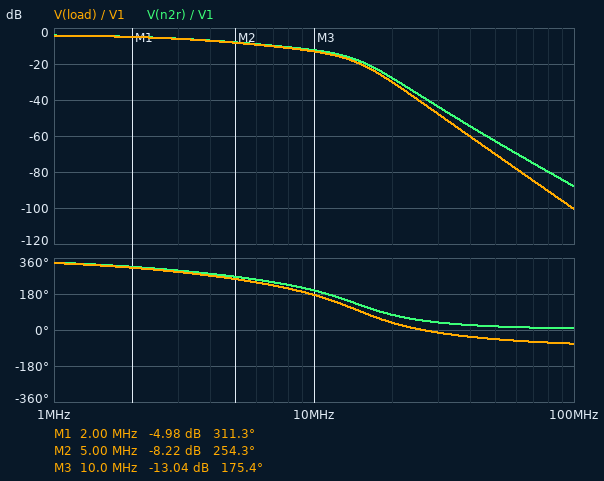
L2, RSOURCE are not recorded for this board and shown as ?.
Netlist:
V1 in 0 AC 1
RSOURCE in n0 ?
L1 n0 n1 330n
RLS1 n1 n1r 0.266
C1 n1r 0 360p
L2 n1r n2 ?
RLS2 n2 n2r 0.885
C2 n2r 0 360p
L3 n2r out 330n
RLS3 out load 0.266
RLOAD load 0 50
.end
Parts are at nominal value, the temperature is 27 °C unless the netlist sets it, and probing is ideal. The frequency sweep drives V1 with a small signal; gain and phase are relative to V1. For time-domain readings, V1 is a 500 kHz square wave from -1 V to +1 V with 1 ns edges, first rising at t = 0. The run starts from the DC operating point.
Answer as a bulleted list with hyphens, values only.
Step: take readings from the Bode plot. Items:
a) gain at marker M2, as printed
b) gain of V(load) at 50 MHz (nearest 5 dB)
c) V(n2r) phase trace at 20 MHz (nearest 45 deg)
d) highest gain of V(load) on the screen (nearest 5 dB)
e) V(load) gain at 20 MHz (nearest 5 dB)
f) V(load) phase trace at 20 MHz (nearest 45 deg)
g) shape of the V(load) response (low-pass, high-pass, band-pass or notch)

- -8.22 dB
- -70 dB
- 90 deg
- -5 dB
- -30 dB
- 45 deg
- low-pass
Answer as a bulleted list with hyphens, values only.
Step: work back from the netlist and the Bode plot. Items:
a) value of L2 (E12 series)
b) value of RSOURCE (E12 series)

- 3.9 µH
- 27 Ω
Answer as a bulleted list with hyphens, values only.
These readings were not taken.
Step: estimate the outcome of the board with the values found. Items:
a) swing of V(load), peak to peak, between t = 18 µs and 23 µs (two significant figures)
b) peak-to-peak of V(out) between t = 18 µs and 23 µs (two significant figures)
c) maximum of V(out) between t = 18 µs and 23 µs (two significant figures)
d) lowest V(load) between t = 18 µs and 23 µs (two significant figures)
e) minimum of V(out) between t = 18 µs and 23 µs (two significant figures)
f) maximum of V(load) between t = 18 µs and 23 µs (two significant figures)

- 1.3 V
- 1.3 V
- 640 mV
- -640 mV
- -640 mV
- 640 mV
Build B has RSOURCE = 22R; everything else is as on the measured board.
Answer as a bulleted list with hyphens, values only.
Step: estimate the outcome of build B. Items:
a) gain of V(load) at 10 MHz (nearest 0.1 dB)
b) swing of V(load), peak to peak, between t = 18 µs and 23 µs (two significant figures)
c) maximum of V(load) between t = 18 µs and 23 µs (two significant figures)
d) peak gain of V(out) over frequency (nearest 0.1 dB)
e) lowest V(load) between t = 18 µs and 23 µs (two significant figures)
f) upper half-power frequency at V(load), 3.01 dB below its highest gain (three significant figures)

- -12.4 dB
- 1.4 V
- 680 mV
- -3.3 dB
- -680 mV
- 3.51 MHz
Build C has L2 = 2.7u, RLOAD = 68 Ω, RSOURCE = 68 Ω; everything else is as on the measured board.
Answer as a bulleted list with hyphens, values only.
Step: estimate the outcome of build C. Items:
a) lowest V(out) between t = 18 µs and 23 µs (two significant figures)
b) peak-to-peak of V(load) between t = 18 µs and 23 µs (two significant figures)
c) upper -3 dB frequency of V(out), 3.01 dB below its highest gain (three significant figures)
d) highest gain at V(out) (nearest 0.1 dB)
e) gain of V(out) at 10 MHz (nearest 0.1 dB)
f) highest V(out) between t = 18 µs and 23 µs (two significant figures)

- -590 mV
- 1.2 V
- 8.16 MHz
- -6.1 dB
- -12.8 dB
- 590 mV
